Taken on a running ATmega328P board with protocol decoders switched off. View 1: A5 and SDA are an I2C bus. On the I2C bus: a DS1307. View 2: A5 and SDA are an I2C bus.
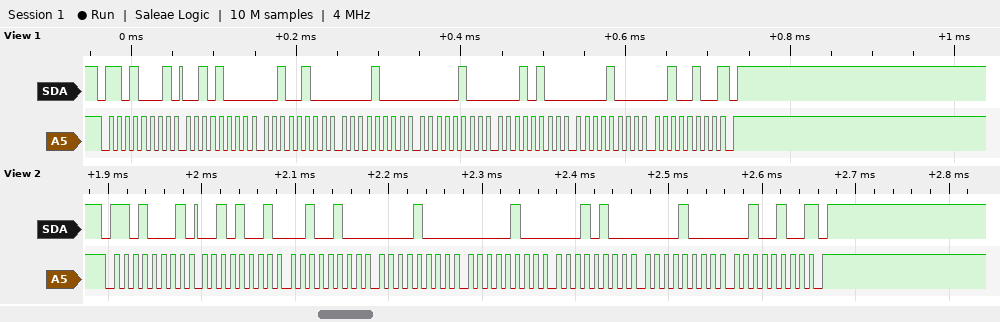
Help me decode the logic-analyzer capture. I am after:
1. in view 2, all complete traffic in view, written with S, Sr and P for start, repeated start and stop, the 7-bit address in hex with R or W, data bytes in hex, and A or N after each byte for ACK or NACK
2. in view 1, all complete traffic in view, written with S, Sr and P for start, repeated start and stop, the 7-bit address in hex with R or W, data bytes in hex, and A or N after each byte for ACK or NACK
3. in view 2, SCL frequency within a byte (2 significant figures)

S 68R A 29 A 24 A 08 A 04 A 14 A 08 A 24 N P
S 68R A 28 A 24 A 08 A 04 A 14 A 08 A 24 N P
100 kHz
